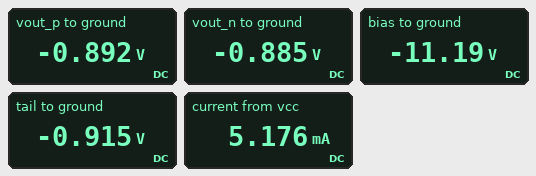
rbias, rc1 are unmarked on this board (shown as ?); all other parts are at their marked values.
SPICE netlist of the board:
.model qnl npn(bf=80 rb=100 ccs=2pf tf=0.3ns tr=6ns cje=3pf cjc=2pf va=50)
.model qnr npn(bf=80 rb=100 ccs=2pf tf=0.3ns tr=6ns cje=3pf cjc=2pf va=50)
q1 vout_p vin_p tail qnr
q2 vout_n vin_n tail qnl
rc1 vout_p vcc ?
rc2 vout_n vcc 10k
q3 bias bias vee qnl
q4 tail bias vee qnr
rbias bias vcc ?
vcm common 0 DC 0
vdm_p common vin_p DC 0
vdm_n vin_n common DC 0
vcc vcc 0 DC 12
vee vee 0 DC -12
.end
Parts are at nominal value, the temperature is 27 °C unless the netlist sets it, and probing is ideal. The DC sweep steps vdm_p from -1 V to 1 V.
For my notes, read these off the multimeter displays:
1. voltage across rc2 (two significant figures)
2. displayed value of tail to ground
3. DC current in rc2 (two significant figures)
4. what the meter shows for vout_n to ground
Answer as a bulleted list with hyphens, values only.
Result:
- 13 V
- -0.915 V
- 1.3 mA
- -0.885 V
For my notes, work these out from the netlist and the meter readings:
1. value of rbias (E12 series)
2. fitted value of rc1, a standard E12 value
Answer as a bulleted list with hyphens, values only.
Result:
- 6.8 kΩ
- 27 kΩ
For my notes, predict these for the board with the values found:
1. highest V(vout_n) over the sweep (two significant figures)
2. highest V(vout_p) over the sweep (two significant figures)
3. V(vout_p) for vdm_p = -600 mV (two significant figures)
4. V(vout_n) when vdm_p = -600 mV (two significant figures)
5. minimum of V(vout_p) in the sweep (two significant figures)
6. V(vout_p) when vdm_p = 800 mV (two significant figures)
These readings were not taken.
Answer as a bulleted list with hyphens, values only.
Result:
- 12 V
- 12 V
- -560 mV
- 12 V
- -980 mV
- 12 V
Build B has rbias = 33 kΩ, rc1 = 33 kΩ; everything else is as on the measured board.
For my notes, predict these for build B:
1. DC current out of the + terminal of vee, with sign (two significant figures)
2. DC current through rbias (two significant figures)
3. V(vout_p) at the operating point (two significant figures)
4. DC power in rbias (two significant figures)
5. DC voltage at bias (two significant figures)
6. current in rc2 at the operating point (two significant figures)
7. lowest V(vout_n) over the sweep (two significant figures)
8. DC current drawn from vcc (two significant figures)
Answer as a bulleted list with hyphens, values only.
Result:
- -1.5 mA
- 700 µA
- -520 mV
- 16 mW
- -11 V
- 440 µA
- 3.8 V
- 1.5 mA
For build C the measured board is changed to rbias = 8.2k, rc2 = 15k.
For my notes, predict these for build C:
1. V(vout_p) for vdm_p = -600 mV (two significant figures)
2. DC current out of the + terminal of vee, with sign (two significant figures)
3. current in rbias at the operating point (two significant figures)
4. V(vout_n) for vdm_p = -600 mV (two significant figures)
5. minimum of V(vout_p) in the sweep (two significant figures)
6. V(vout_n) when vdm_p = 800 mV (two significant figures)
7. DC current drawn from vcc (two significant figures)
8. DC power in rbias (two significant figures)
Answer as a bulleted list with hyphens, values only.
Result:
- -490 mV
- -6.2 mA
- 2.8 mA
- 12 V
- -950 mV
- -1.0 V
- 4.2 mA
- 66 mW
